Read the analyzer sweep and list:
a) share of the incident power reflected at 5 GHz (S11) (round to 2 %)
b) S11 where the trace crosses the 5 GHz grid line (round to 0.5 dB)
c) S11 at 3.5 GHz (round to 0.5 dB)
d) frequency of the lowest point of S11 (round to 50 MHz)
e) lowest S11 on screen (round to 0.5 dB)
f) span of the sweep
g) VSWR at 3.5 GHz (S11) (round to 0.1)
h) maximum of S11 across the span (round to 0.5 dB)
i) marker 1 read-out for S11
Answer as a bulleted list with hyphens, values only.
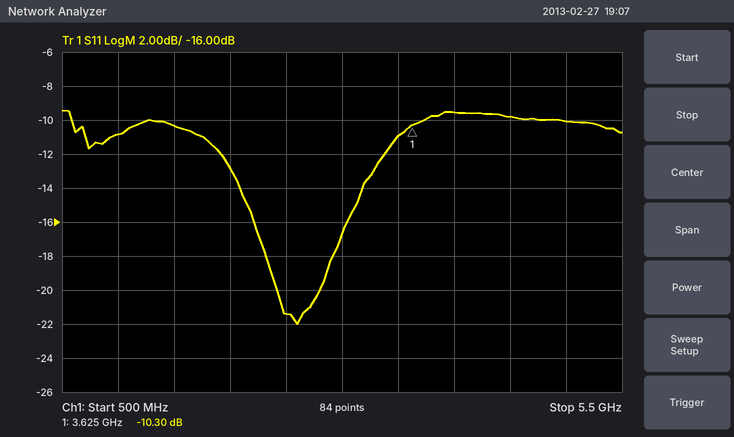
- 10 %
- -10.0 dB
- -11.0 dB
- 2.60 GHz
- -22.0 dB
- 5 GHz
- 1.8
- -9.5 dB
- -10.30 dB
